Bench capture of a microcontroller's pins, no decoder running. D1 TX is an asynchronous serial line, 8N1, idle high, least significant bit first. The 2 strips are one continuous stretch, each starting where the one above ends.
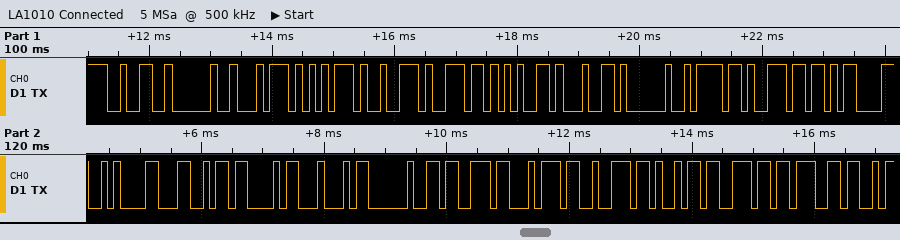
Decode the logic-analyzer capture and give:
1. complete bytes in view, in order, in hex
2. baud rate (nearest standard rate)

0x32 0x20 0x74 0x75 0x72 0x6E 0x65 0x64 0x20 0x6F 0x6E 0x0D 0x0A 0x4C 0x43 0x44 0x20 0x73 0x74 0x72 0x69 0x6E 0x67
9600 baud
